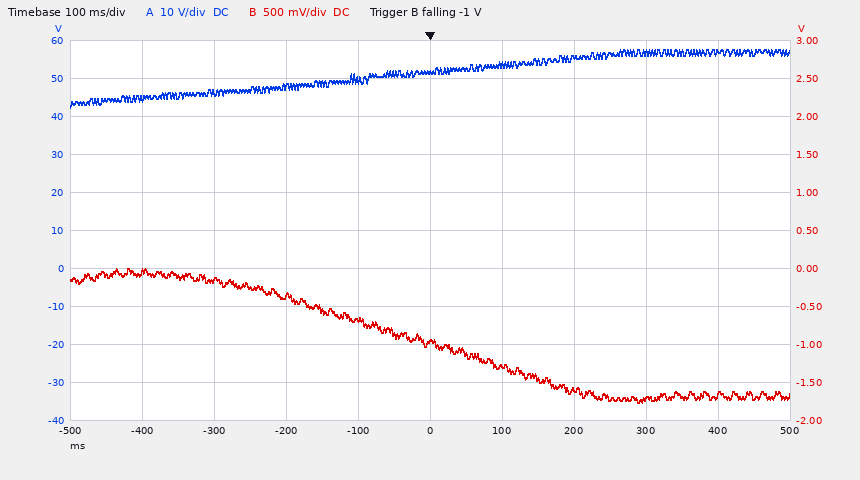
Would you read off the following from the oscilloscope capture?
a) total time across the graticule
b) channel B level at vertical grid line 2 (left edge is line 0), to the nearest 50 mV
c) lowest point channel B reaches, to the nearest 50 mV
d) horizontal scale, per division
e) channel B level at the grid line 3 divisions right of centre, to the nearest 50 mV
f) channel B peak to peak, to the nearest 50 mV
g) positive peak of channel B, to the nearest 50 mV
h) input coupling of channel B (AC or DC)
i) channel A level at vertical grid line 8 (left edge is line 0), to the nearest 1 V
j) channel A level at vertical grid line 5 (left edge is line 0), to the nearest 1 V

1 s
-150 mV
-1.75 V
100 ms
-1.70 V
1.75 V
0 mV
DC
57 V
52 V
